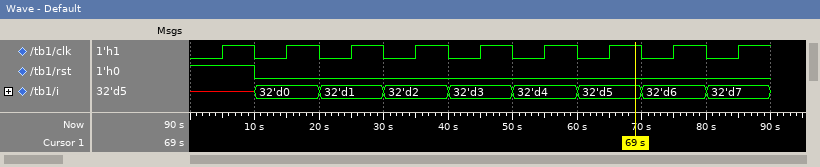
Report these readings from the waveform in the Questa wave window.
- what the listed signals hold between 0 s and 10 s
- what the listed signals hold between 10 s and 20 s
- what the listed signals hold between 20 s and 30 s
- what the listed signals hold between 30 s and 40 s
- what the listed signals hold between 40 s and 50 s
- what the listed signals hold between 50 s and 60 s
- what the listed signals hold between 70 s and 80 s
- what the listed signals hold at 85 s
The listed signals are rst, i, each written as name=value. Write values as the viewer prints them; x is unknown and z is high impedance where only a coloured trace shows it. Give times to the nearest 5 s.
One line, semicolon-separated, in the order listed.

rst=1, i=x; rst=0, i=32'd0; rst=0, i=32'd1; rst=0, i=32'd2; rst=0, i=32'd3; rst=0, i=32'd4; rst=0, i=32'd6; rst=0, i=32'd7
